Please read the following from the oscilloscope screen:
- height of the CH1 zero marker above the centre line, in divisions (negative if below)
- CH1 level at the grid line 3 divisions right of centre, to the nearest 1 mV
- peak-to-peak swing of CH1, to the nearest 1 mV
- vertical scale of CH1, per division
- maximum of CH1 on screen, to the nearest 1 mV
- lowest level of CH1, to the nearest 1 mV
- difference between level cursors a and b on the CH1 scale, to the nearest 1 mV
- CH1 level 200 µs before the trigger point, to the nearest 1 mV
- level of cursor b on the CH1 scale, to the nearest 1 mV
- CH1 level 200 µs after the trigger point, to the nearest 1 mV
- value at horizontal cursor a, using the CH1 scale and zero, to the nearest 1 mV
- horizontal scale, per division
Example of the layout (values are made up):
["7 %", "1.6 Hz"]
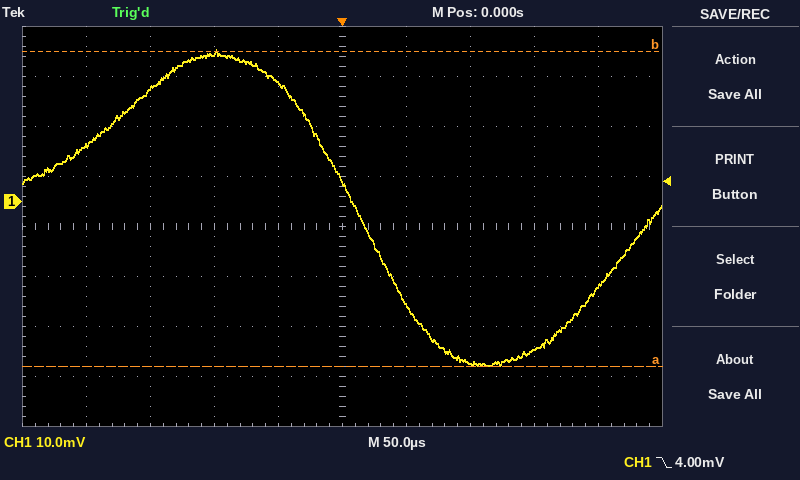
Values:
["+0.5 div", "-30 mV", "63 mV", "10 mV", "30 mV", "-33 mV", "63 mV", "11 mV", "30 mV", "-17 mV", "-33 mV", "50 µs"]
